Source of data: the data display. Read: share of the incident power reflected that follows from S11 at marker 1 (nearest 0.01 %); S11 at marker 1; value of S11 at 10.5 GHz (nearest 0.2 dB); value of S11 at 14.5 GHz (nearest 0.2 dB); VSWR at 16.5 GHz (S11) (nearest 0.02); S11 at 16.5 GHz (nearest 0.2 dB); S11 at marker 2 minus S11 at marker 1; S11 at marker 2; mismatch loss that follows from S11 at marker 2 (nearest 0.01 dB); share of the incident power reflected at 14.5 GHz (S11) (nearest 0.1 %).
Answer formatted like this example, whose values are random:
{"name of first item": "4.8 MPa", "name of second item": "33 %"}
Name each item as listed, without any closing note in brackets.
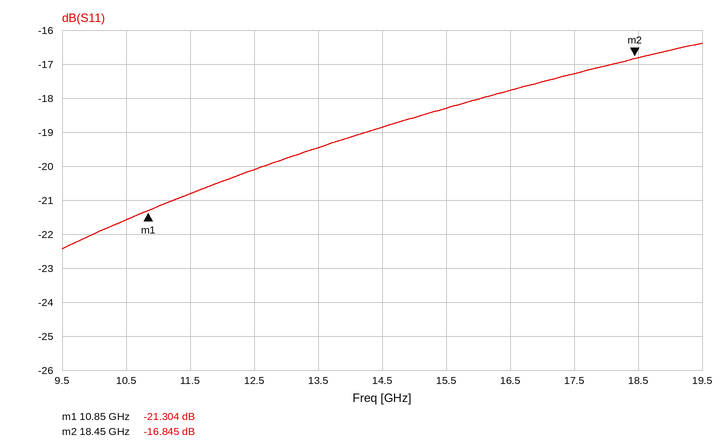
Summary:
{"share of the incident power reflected that follows from S11 at marker 1": "0.74 %", "S11 at marker 1": "-21.304 dB", "value of S11 at 10.5 GHz": "-21.6 dB", "value of S11 at 14.5 GHz": "-18.8 dB", "VSWR at 16.5 GHz (S11)": "1.30", "S11 at 16.5 GHz": "-17.8 dB", "S11 at marker 2 minus S11 at marker 1": "4.459 dB", "S11 at marker 2": "-16.845 dB", "mismatch loss that follows from S11 at marker 2": "0.09 dB", "share of the incident power reflected at 14.5 GHz (S11)": "1.3 %"}
